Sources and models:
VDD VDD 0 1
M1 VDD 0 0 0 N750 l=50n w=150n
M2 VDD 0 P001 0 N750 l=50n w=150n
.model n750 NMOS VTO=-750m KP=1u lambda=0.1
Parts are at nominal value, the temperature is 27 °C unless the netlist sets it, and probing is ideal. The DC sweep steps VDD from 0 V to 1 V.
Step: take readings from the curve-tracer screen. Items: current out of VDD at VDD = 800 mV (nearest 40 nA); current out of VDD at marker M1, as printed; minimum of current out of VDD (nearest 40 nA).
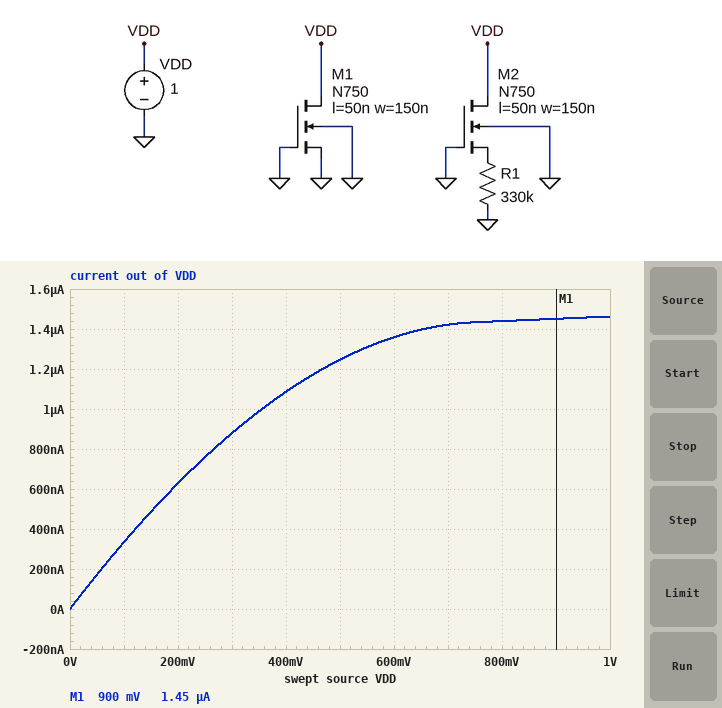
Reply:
1.44 µA
1.45 µA
0 A
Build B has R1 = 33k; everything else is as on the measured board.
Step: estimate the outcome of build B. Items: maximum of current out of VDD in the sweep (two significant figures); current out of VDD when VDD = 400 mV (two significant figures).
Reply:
1.8 µA
1.3 µA
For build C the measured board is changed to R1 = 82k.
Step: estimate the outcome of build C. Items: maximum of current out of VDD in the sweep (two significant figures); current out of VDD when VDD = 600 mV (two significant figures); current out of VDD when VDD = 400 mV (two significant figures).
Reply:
1.7 µA
1.6 µA
1.3 µA
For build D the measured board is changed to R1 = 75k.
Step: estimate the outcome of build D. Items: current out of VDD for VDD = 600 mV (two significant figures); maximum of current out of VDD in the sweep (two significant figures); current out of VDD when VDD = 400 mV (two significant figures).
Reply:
1.6 µA
1.7 µA
1.3 µA
